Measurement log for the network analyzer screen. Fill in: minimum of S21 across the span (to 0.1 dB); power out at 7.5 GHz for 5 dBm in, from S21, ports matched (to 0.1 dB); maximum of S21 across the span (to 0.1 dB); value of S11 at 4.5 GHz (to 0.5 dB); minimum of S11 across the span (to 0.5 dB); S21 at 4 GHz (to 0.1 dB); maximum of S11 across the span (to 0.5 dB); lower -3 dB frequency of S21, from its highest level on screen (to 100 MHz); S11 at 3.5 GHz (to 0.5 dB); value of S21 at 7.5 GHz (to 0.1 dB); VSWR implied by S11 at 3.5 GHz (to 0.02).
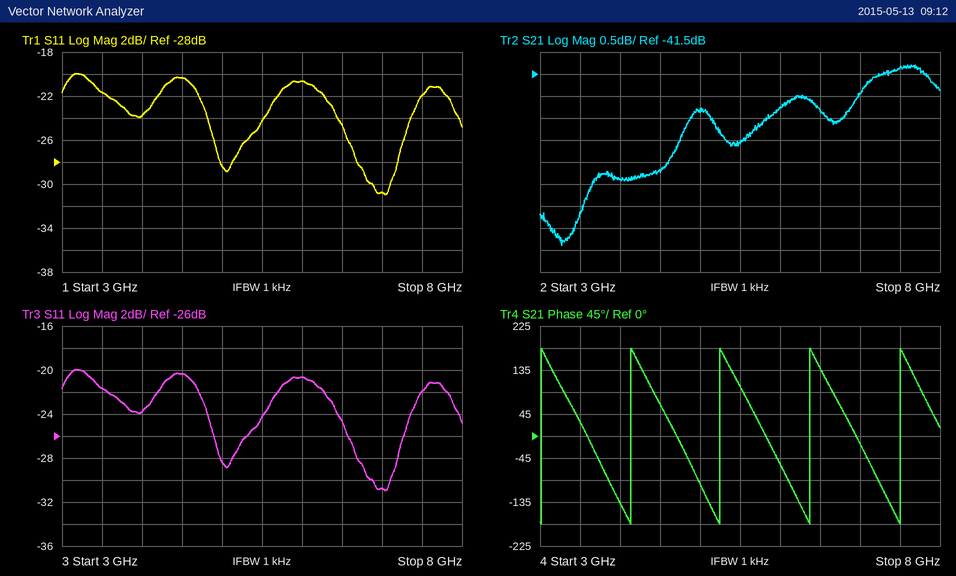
-45.4 dB
-36.3 dBm
-41.3 dB
-20.5 dB
-31.0 dB
-43.9 dB
-20.0 dB
3.6 GHz
-21.5 dB
-41.3 dB
1.18
